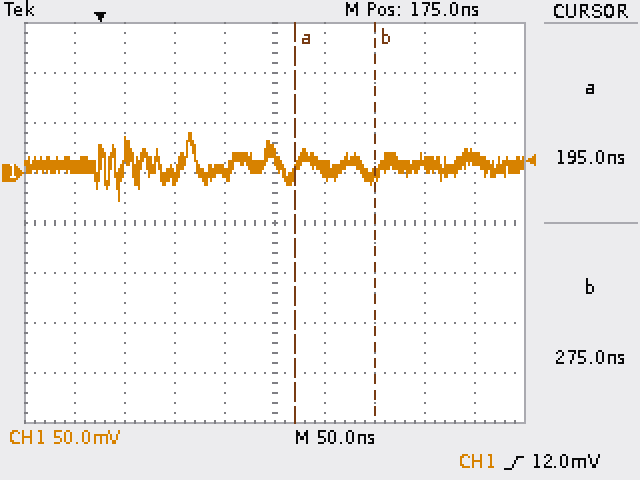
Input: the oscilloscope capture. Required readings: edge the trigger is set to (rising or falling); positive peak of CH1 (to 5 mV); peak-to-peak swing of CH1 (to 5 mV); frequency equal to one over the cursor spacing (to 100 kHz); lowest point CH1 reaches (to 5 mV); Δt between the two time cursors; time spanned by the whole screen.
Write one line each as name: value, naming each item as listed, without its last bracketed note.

edge the trigger is set to: rising
positive peak of CH1: 40 mV
peak-to-peak swing of CH1: 70 mV
frequency equal to one over the cursor spacing: 12.5 MHz
lowest point CH1 reaches: -30 mV
Δt between the two time cursors: 80 ns
time spanned by the whole screen: 500 ns
